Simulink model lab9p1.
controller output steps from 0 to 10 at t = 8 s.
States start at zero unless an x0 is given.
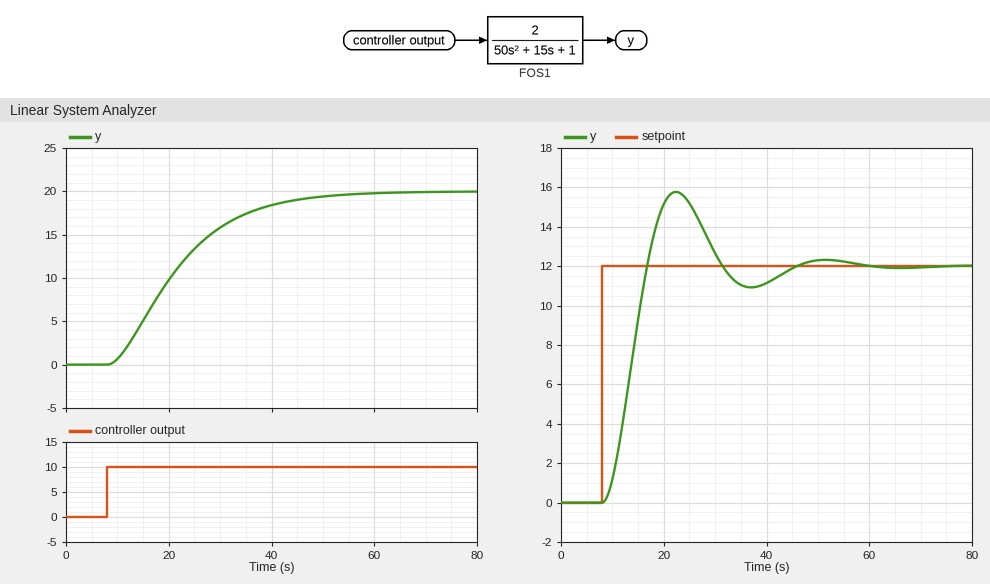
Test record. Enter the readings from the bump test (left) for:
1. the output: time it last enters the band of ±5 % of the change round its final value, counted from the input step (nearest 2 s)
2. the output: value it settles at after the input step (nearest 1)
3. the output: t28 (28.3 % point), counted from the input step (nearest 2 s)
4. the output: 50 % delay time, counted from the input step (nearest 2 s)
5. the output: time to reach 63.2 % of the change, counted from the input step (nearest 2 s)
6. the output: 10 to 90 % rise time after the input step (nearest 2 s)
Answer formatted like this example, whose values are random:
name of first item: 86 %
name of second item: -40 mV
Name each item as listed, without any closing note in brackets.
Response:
the output: time it last enters the band of ±5 % of the change round its final value, counted from the input step: 36 s
the output: value it settles at after the input step: 20
the output: t28 (28.3 % point), counted from the input step: 8 s
the output: 50 % delay time, counted from the input step: 12 s
the output: time to reach 63.2 % of the change, counted from the input step: 16 s
the output: 10 to 90 % rise time after the input step: 26 s
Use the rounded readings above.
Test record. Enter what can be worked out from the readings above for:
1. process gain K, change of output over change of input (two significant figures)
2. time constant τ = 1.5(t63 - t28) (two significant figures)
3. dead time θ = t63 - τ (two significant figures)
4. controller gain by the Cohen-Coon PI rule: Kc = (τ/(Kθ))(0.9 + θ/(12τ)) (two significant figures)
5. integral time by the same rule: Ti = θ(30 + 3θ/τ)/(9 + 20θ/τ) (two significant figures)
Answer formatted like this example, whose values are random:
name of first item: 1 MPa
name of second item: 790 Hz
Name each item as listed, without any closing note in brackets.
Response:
process gain K, change of output over change of input: 2.0
time constant τ = 1.5(t63 - t28): 12 s
dead time θ = t63 - τ: 4.0 s
controller gain by the Cohen-Coon PI rule: Kc = (τ/(Kθ))(0.9 + θ/(12τ)): 1.4
integral time by the same rule: Ti = θ(30 + 3θ/τ)/(9 + 20θ/τ): 7.9 s
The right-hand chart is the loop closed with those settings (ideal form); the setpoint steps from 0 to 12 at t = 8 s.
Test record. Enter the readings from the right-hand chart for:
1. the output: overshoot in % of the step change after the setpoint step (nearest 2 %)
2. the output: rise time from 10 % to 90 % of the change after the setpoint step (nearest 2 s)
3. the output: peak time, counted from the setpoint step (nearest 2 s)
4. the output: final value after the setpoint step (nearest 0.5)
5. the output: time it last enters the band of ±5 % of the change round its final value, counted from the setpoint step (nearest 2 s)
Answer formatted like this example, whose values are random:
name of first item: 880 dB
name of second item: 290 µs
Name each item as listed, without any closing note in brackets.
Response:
the output: overshoot in % of the step change after the setpoint step: 32 %
the output: rise time from 10 % to 90 % of the change after the setpoint step: 6 s
the output: peak time, counted from the setpoint step: 14 s
the output: final value after the setpoint step: 12.0
the output: time it last enters the band of ±5 % of the change round its final value, counted from the setpoint step: 34 s
